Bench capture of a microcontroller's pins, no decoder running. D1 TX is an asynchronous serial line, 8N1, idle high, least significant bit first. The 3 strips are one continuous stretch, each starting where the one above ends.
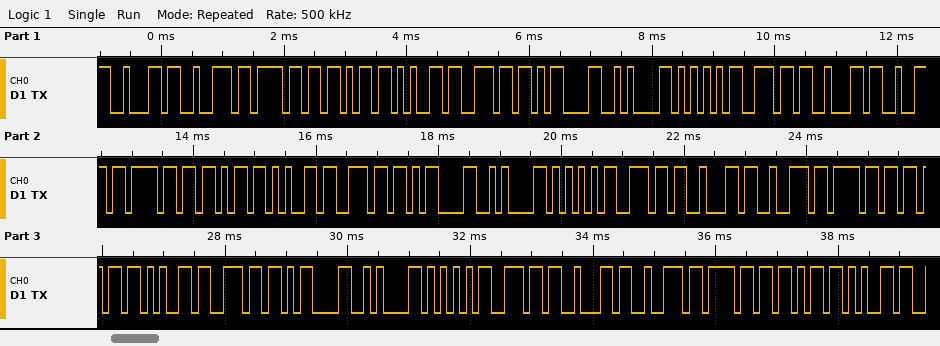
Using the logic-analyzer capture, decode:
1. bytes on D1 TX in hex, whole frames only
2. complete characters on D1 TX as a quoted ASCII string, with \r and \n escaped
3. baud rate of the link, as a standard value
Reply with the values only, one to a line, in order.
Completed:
62 72 6F 6B 65 6E 0D 0A 55 6E 62 72 6F 6B 65 6E 0D 0A 55 6E 62 72 6F 6B 65 6E 0D 0A 55 6E 62 72 6F 6B 65
"broken\r\nUnbroken\r\nUnbroken\r\nUnbroke"
9600 baud
